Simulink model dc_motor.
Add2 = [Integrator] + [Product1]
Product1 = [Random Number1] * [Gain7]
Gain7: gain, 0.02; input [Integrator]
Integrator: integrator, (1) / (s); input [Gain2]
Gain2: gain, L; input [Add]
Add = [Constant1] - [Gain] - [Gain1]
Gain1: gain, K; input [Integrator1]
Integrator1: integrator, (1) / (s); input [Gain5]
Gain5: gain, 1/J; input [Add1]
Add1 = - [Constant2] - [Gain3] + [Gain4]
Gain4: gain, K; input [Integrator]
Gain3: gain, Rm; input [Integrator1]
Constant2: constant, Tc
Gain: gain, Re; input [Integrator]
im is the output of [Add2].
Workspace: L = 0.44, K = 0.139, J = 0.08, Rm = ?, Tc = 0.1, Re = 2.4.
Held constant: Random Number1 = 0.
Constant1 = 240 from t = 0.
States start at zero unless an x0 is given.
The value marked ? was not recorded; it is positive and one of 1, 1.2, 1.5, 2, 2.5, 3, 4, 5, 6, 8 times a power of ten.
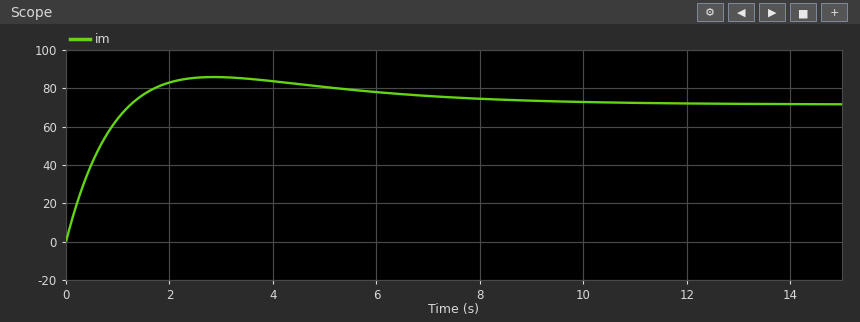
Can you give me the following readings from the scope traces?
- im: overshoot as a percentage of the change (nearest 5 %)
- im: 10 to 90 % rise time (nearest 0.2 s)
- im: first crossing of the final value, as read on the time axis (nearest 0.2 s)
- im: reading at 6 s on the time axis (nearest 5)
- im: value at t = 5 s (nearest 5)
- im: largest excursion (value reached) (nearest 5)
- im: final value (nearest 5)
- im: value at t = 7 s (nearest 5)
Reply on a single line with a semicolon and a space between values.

20 %; 1.0 s; 1.2 s; 80; 80; 85; 70; 75
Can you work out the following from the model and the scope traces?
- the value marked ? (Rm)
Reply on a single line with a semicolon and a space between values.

0.02
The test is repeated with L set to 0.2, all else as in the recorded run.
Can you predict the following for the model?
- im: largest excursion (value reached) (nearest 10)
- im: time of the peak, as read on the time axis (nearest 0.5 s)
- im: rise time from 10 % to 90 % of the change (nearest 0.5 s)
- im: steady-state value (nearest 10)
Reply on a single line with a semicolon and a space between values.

80; 5.5 s; 2.0 s; 70
